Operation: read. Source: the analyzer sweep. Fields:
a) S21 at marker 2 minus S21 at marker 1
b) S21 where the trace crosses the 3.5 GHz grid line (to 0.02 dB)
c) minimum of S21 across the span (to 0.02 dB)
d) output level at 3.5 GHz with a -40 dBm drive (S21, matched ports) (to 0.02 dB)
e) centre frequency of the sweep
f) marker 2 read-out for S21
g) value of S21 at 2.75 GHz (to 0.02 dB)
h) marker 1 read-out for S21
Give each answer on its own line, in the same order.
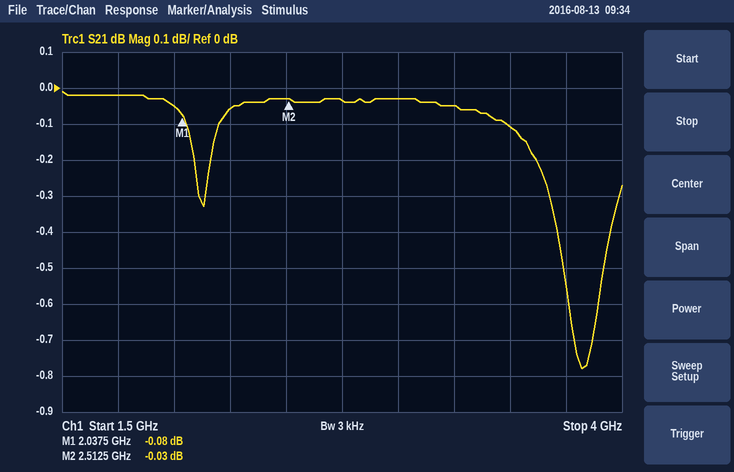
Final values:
0.05 dB
-0.10 dB
-0.78 dB
-40.10 dBm
2.75 GHz
-0.03 dB
-0.04 dB
-0.08 dB
